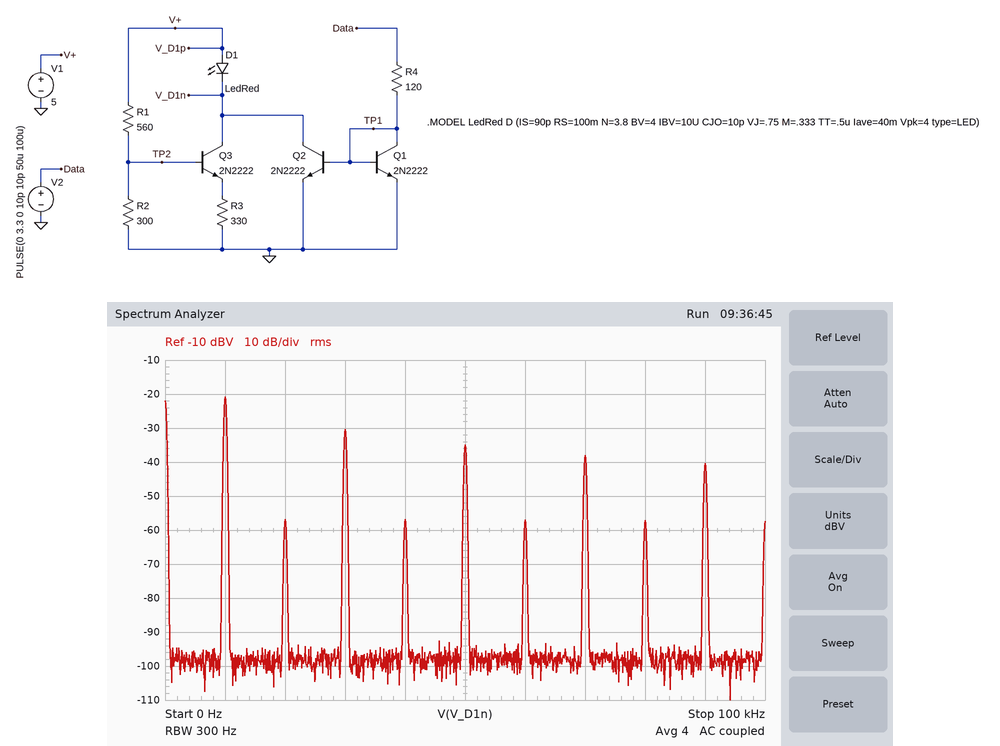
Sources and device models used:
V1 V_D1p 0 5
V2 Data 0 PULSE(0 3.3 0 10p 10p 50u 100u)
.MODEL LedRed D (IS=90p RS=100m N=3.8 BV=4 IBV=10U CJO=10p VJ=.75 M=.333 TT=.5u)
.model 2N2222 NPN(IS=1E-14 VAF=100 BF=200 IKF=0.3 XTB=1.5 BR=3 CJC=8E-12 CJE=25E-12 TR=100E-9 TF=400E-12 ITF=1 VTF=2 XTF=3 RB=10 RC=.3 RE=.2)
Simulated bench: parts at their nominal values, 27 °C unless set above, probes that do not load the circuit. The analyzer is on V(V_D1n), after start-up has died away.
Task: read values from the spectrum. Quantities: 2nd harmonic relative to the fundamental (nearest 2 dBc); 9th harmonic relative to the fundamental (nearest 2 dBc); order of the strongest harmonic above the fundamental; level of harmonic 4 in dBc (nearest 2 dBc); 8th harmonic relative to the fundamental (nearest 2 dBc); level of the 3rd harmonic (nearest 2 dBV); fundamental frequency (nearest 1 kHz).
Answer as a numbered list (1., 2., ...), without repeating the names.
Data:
1. -36 dBc
2. -20 dBc
3. 3
4. -36 dBc
5. -36 dBc
6. -30 dBV
7. 10 kHz
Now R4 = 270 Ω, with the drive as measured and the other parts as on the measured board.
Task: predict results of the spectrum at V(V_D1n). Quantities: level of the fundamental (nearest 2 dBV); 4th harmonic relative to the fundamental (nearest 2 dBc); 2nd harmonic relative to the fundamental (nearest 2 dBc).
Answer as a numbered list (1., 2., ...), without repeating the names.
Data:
1. -24 dBV
2. -40 dBc
3. -40 dBc
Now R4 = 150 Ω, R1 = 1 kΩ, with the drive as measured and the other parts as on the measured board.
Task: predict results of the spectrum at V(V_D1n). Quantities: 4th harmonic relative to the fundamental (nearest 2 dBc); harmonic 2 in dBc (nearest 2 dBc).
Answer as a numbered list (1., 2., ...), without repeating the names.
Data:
1. -34 dBc
2. -34 dBc
